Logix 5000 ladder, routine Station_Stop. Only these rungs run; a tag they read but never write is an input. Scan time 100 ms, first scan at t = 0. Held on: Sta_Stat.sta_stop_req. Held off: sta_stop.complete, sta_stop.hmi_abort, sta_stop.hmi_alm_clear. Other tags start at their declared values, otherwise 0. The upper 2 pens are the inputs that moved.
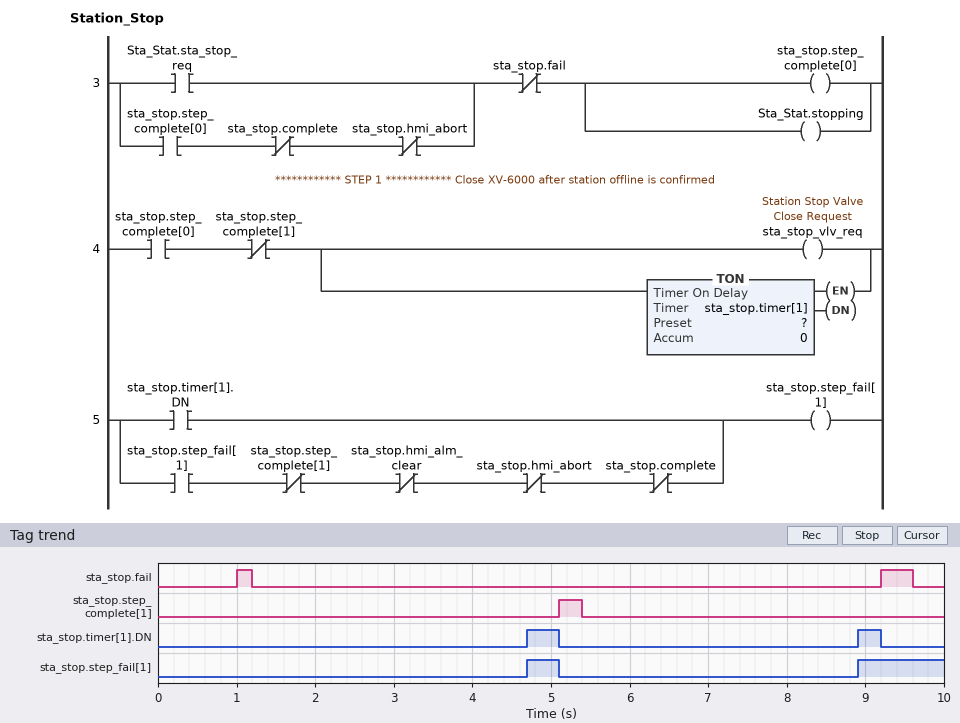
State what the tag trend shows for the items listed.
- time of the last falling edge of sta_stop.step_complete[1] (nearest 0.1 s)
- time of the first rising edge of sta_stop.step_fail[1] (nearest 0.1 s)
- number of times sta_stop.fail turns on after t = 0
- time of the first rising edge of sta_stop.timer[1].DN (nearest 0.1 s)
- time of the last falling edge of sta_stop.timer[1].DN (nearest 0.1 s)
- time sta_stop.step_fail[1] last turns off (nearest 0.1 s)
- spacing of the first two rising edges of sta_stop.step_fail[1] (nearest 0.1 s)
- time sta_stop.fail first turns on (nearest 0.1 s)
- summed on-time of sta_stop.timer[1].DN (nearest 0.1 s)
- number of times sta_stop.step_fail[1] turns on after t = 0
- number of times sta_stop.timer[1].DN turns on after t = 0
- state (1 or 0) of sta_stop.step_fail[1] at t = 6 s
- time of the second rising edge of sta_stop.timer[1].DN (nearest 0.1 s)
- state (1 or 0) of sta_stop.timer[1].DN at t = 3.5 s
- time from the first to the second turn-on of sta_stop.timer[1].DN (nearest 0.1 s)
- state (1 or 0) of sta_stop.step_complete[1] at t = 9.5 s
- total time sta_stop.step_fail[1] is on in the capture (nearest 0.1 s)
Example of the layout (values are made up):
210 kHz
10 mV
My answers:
5.4 s
4.7 s
2
4.7 s
9.2 s
5.1 s
4.2 s
1.0 s
0.7 s
2
2
0
8.9 s
0
4.2 s
0
1.5 s
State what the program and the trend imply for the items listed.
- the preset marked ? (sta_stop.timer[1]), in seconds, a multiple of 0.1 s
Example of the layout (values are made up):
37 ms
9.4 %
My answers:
3.5 s
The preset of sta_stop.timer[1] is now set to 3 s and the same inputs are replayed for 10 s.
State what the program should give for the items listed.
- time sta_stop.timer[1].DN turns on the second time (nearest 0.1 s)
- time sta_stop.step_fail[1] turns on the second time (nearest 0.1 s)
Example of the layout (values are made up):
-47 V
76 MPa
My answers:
8.4 s
8.4 s
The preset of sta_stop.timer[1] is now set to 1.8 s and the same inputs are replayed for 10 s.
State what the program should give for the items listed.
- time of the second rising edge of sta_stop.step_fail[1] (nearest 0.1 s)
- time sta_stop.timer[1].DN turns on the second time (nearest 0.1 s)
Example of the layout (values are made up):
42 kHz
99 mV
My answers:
7.2 s
7.2 s
